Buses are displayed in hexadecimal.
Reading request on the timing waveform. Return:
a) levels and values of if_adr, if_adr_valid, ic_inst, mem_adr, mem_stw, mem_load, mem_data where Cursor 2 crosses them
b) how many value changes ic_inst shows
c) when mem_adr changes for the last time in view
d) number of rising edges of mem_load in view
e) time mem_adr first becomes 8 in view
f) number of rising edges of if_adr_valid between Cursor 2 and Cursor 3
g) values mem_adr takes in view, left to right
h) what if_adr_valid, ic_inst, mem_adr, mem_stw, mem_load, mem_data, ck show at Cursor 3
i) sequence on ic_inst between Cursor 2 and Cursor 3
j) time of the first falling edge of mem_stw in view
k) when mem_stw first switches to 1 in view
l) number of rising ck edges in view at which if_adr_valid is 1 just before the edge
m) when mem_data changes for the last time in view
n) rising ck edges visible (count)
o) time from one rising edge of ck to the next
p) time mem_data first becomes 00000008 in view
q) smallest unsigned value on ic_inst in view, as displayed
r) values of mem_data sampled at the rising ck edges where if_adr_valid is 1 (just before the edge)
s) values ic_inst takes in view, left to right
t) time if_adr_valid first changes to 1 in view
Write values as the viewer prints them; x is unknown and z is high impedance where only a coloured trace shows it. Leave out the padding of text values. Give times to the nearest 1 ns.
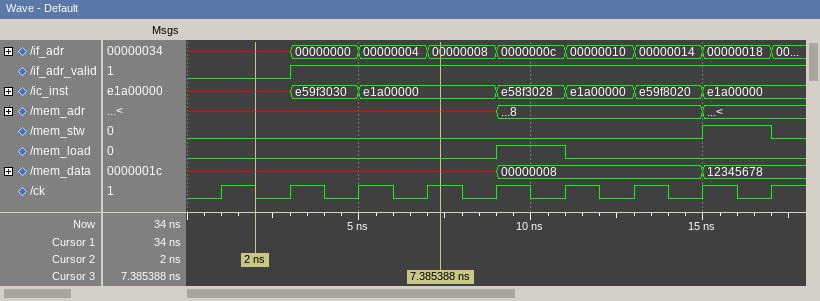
if_adr=x, if_adr_valid=0, ic_inst=x, mem_adr=x, mem_stw=0, mem_load=0, mem_data=x
6
15 ns
1
9 ns
1
x, 8, <
if_adr_valid=1, ic_inst=e1a00000, mem_adr=x, mem_stw=0, mem_load=0, mem_data=x, ck=1
x, e59f3030, e1a00000
17 ns
15 ns
7
15 ns
9
2 ns
9 ns
e1a00000
x, x, x, 00000008, 00000008, 00000008, 12345678
x, e59f3030, e1a00000, e58f3028, e1a00000, e59f8020, e1a00000
3 ns
